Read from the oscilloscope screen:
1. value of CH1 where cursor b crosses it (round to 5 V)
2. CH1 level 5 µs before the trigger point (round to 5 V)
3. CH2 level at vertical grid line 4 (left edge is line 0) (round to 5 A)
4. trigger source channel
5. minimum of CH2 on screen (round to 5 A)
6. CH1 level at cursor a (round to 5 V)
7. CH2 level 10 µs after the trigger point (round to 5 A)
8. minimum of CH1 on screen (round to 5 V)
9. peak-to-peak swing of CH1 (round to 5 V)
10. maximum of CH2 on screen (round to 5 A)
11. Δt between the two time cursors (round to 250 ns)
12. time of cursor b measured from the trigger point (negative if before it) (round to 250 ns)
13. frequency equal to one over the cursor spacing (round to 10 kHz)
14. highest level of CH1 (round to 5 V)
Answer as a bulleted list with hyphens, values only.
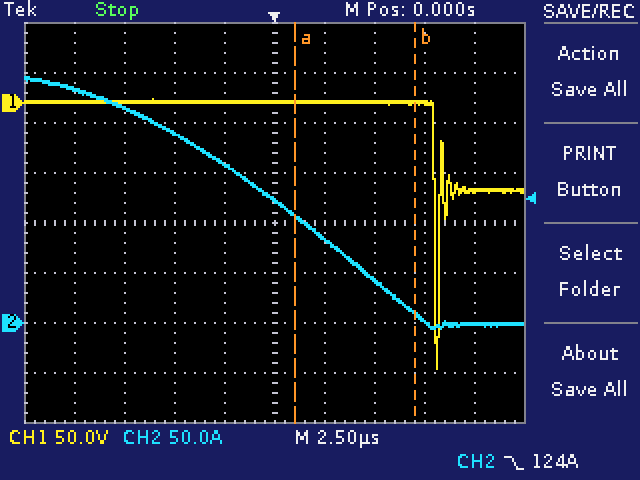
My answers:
- 0 V
- 0 V
- 160 A
- CH2
- -5 A
- 0 V
- 0 A
- -265 V
- 270 V
- 245 A
- 6.00 µs
- +7.00 µs
- 170 kHz
- 5 V
